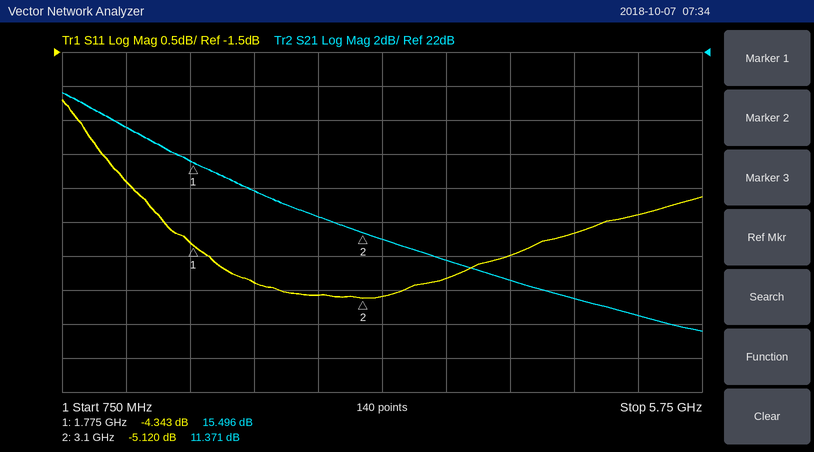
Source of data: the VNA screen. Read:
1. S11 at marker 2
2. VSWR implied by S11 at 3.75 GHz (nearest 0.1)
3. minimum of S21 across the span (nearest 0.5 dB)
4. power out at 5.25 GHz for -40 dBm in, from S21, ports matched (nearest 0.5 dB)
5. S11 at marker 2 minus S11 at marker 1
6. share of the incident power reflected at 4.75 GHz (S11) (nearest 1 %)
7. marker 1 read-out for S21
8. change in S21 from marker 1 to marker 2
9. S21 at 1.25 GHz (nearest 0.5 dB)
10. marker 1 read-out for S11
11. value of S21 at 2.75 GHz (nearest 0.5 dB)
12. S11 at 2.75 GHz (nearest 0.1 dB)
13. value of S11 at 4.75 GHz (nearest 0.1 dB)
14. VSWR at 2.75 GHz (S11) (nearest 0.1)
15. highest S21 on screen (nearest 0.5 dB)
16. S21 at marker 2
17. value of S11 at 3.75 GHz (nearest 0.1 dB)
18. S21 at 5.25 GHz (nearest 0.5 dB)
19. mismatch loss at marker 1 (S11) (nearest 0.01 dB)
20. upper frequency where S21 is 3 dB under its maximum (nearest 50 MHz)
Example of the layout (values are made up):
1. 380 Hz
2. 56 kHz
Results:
1. -5.120 dB
2. 3.7
3. 5.5 dB
4. -33.5 dBm
5. -0.777 dB
6. 38 %
7. 15.496 dB
8. -4.125 dB
9. 17.5 dB
10. -4.343 dB
11. 12.5 dB
12. -5.1 dB
13. -4.2 dB
14. 3.5
15. 19.5 dB
16. 11.371 dB
17. -4.8 dB
18. 6.5 dB
19. 1.99 dB
20. 1.50 GHz
